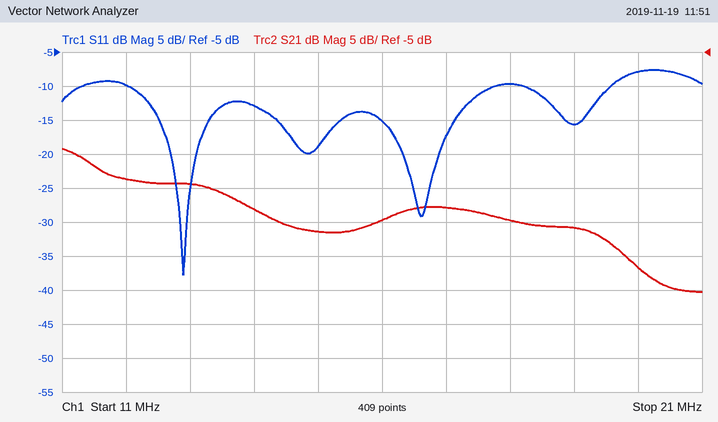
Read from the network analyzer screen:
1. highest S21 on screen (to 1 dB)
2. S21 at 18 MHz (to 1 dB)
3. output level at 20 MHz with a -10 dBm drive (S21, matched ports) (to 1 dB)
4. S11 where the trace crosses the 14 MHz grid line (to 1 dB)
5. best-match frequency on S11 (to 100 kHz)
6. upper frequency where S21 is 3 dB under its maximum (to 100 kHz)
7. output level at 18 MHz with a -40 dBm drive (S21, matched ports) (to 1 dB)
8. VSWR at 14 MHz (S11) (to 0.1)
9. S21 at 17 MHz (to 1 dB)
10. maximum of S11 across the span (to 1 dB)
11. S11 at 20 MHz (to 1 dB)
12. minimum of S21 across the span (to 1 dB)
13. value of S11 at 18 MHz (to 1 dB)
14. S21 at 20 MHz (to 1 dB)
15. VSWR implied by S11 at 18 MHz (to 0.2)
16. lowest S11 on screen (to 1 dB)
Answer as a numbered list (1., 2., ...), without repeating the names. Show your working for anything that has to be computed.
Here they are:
1. -19 dB
2. -30 dB
3. -10 dBm + (-37 dB) = -47 dBm
4. -13 dB
5. 12.9 MHz
6. 11.6 MHz
7. -40 dBm + (-30 dB) = -70 dBm
8. |Γ| = 10^(-13/20) = 0.2239; VSWR = (1 + 0.2239)/(1 − 0.2239) ≈ 1.6
9. -28 dB
10. -8 dB
11. -8 dB
12. -40 dB
13. -10 dB
14. -37 dB
15. |Γ| = 10^(-10/20) = 0.3162; VSWR = (1 + 0.3162)/(1 − 0.3162) ≈ 1.92, so 2.0 to the nearest 0.2
16. -38 dB
